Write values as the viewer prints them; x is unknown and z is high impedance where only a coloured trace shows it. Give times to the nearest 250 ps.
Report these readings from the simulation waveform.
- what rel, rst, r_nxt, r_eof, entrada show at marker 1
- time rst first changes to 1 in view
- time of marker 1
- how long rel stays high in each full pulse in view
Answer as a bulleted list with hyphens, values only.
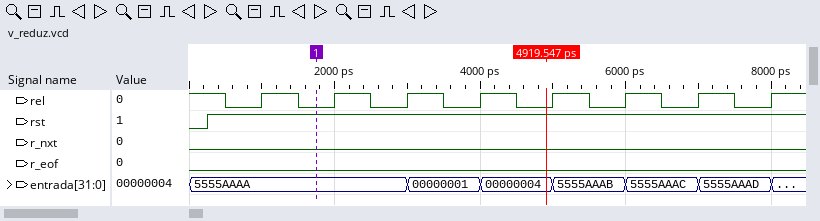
- rel=0, rst=1, r_nxt=0, r_eof=0, entrada=5555AAAA
- 250 ps
- 1750 ps
- 500 ps, 500 ps, 500 ps, 500 ps, 500 ps, 500 ps, 500 ps
